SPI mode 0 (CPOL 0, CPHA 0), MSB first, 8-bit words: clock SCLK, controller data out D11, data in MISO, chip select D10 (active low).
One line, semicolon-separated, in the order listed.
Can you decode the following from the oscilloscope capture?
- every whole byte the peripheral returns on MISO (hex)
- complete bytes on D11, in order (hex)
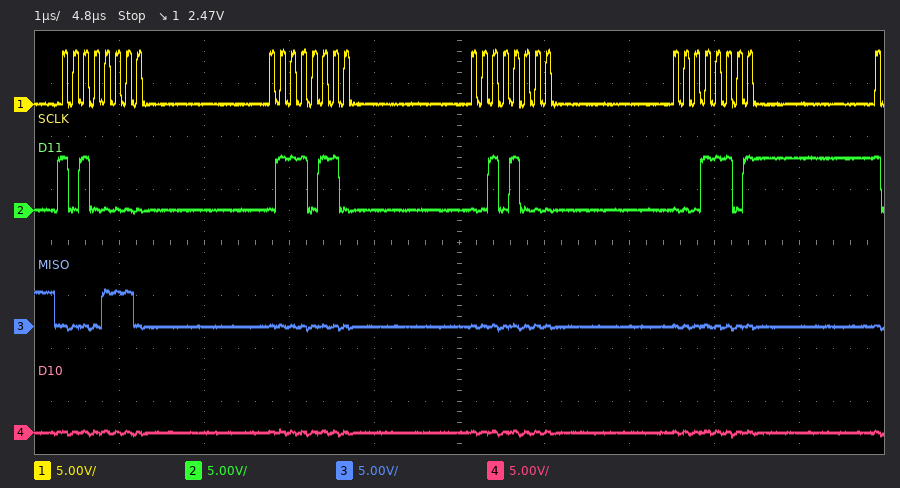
0E 00 00 00; A0 76 28 1D
